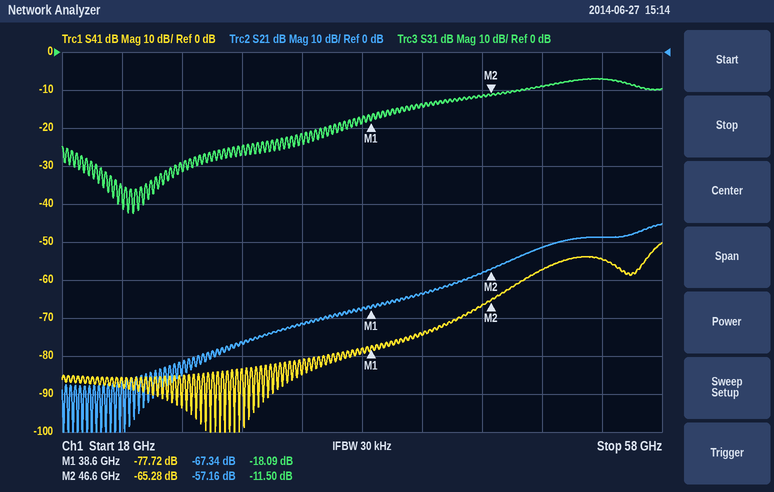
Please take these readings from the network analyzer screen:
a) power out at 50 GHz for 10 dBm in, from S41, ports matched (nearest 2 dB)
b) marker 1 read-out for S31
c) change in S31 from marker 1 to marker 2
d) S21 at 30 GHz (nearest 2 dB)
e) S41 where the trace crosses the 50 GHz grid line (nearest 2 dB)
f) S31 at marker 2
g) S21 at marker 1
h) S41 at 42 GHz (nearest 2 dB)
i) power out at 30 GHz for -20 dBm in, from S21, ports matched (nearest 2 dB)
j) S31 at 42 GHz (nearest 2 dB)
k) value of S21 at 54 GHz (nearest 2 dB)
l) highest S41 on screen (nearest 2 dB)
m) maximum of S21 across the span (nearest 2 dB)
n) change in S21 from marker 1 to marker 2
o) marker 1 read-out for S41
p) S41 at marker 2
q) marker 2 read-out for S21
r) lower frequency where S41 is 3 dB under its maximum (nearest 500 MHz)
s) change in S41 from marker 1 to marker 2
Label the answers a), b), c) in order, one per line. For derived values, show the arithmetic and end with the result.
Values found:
a) 10 dBm + (-58 dB) = -48 dBm
b) -18.09 dB
c) -11.5 − (-18.09) = 6.59 dB
d) -76 dB
e) -58 dB
f) -11.50 dB
g) -67.34 dB
h) -74 dB
i) -20 dBm + (-76 dB) = -96 dBm
j) -14 dB
k) -48 dB
l) -50 dB
m) -46 dB
n) -57.16 − (-67.34) = 10.18 dB
o) -77.72 dB
p) -65.28 dB
q) -57.16 dB
r) 57.0 GHz
s) -65.28 − (-77.72) = 12.44 dB
